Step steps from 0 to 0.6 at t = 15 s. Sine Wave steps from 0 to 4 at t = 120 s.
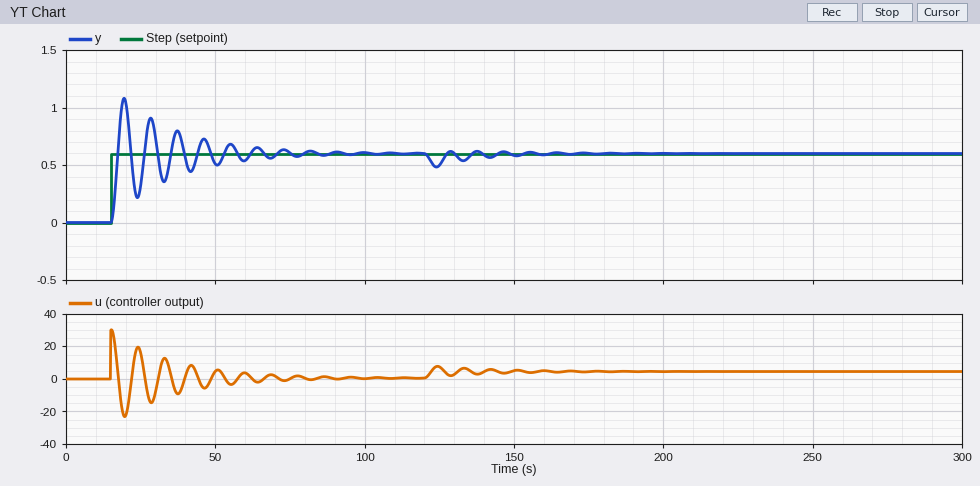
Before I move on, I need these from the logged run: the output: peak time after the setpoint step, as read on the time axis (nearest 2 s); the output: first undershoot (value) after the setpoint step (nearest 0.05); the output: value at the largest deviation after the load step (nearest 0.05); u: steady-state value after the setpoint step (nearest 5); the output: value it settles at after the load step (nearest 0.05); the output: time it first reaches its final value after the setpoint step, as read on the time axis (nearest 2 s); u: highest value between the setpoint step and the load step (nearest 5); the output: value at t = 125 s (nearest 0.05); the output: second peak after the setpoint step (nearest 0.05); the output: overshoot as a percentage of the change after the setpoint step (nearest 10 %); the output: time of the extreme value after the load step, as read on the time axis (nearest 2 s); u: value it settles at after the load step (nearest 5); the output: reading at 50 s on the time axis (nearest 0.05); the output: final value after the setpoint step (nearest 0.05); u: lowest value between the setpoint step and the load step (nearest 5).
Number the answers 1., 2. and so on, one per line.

1. 20 s
2. 0.20
3. 0.50
4. 0
5. 0.60
6. 18 s
7. 30
8. 0.50
9. 0.90
10. 80 %
11. 124 s
12. 5
13. 0.50
14. 0.60
15. -25
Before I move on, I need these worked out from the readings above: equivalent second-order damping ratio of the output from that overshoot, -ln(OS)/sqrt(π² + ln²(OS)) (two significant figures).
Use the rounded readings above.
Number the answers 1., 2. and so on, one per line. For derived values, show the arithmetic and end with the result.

1. ln(0.8) = -0.223; 0.223 / sqrt(9.870 + 0.050) = 0.071
